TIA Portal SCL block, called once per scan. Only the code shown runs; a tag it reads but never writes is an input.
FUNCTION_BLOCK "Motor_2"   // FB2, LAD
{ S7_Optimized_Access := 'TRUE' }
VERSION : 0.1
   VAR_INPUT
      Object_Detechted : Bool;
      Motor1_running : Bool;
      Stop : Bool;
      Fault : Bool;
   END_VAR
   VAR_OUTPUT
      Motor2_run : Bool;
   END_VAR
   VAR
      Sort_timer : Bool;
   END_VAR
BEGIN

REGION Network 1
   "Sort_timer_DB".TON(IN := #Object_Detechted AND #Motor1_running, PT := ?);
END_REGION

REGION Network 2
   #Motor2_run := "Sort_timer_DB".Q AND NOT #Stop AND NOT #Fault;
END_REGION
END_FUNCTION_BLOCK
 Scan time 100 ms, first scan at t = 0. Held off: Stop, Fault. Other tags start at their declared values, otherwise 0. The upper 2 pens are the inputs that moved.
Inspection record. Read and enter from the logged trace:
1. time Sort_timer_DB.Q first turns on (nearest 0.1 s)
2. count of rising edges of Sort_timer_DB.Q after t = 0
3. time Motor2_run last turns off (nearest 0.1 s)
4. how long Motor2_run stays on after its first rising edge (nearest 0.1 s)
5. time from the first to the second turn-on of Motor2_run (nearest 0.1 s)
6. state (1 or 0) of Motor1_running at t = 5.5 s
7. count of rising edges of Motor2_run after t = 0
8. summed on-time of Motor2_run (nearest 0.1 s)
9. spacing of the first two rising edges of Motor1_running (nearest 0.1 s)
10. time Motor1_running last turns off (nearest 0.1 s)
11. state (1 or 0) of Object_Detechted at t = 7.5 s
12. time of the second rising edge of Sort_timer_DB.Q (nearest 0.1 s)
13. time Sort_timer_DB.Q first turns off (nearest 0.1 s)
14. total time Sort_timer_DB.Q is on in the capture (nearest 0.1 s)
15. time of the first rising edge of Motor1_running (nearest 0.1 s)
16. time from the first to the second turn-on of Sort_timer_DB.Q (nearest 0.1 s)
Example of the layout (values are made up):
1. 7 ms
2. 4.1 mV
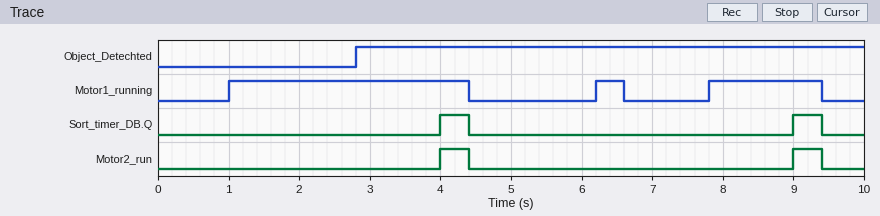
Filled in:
1. 4.0 s
2. 2
3. 9.4 s
4. 0.4 s
5. 5.0 s
6. 0
7. 2
8. 0.8 s
9. 5.2 s
10. 9.4 s
11. 1
12. 9.0 s
13. 4.4 s
14. 0.8 s
15. 1.0 s
16. 5.0 s
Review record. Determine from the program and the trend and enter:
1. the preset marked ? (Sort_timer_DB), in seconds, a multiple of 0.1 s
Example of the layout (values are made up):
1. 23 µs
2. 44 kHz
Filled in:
1. 1.2 s
